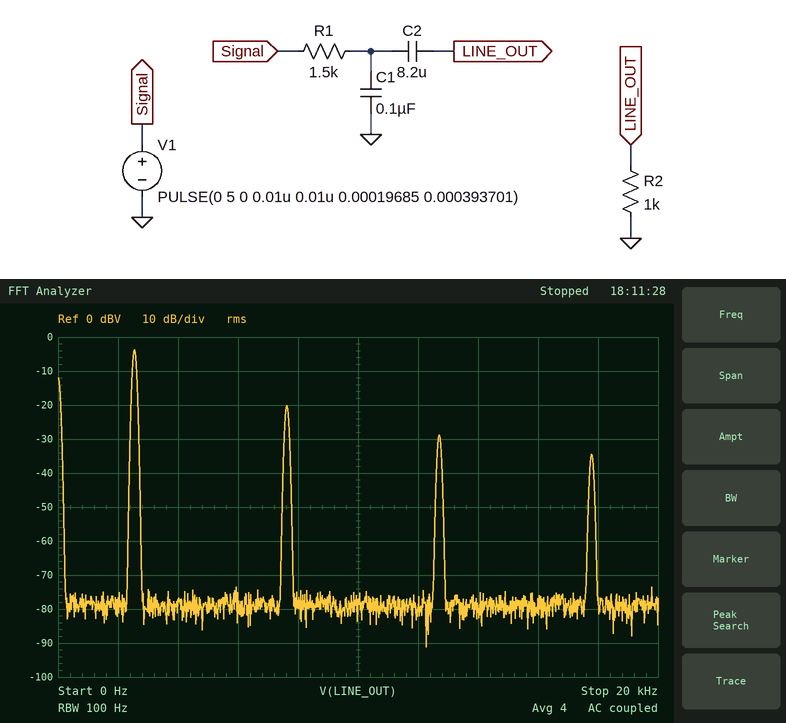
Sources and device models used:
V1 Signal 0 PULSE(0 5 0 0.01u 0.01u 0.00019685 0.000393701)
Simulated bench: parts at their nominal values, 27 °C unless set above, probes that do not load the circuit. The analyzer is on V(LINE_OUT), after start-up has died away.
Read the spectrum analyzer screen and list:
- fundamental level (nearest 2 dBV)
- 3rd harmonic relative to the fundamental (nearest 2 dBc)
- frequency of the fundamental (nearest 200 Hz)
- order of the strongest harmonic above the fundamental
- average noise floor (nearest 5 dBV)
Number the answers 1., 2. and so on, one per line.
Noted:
1. -4 dBV
2. -16 dBc
3. 2.6 kHz
4. 3
5. -80 dBV
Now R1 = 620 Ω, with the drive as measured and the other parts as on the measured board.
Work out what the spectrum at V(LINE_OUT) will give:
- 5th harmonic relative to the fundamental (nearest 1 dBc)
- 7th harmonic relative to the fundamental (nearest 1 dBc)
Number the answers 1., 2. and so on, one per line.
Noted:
1. -23 dBc
2. -28 dBc
